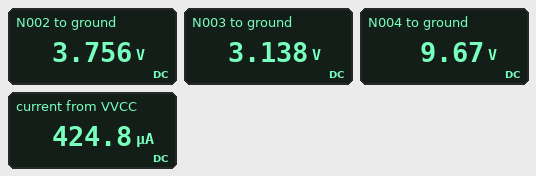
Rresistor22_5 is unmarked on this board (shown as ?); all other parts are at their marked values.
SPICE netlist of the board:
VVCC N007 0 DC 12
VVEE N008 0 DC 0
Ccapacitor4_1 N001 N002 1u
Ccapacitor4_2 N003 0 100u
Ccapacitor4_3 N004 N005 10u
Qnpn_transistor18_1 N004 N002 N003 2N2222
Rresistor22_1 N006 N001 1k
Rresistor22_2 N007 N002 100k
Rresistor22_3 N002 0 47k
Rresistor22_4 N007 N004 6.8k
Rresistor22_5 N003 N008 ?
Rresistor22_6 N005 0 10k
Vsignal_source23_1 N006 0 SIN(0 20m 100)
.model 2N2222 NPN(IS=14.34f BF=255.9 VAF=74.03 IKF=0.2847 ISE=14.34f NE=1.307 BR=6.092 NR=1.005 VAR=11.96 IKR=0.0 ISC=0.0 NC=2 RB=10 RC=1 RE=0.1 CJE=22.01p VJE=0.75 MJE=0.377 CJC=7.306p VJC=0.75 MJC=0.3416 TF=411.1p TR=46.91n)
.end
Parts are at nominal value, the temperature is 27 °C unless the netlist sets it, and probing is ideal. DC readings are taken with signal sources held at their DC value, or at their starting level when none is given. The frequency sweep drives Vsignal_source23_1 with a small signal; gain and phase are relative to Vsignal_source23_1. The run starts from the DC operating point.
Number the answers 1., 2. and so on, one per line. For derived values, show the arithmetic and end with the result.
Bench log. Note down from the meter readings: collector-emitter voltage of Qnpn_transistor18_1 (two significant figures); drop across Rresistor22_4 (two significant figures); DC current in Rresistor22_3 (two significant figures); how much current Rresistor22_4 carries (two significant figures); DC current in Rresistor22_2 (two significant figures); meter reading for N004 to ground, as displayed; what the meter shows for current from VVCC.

1. 9.67 V - 3.138 V = 6.5 V
2. 12 V - 9.67 V = 2.3 V
3. (3.756 V) / 47 kΩ = 80 µA
4. (12 V - 9.67 V) / 6.8 kΩ = 340 µA
5. (12 V - 3.756 V) / 100 kΩ = 82 µA
6. 9.67 V
7. 424.8 µA
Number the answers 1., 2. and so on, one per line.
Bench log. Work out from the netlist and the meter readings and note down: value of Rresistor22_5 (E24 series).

1. 9.1 kΩ
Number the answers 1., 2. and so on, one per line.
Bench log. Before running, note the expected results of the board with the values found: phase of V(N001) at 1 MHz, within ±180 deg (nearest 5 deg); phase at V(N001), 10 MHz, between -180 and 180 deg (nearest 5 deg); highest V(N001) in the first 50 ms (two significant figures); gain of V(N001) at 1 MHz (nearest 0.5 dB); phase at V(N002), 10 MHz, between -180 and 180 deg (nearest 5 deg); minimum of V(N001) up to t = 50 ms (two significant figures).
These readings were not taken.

1. -50 deg
2. -50 deg
3. 18 mV
4. -5.5 dB
5. -50 deg
6. -18 mV
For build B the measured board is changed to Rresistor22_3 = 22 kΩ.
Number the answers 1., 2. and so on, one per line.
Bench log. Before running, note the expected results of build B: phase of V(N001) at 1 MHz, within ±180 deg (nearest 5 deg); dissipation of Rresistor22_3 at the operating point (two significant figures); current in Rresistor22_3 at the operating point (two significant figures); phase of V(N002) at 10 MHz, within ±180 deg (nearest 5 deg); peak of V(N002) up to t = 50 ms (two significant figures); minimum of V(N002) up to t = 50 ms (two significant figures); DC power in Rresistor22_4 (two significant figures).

1. -35 deg
2. 210 µW
3. 97 µA
4. -55 deg
5. 2.2 V
6. 2.1 V
7. 190 µW
